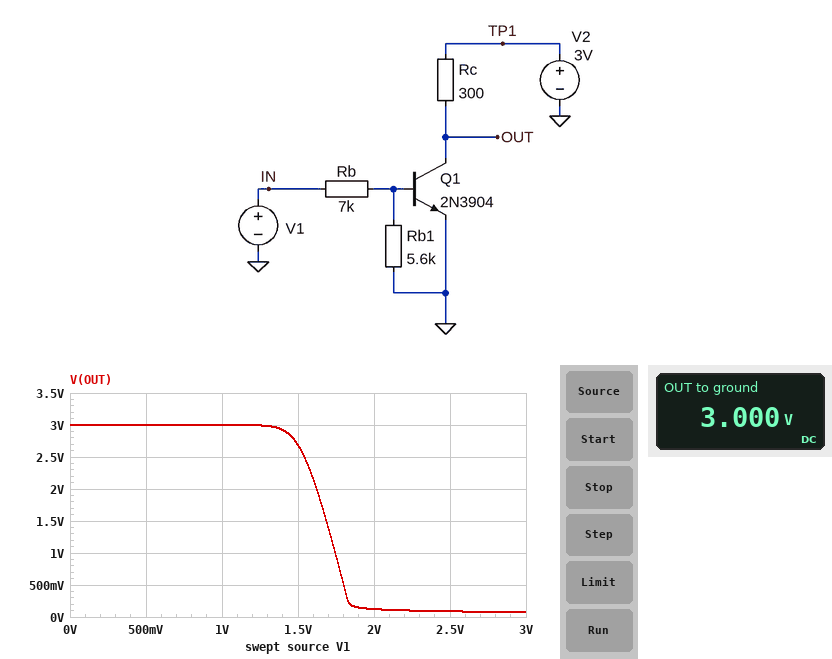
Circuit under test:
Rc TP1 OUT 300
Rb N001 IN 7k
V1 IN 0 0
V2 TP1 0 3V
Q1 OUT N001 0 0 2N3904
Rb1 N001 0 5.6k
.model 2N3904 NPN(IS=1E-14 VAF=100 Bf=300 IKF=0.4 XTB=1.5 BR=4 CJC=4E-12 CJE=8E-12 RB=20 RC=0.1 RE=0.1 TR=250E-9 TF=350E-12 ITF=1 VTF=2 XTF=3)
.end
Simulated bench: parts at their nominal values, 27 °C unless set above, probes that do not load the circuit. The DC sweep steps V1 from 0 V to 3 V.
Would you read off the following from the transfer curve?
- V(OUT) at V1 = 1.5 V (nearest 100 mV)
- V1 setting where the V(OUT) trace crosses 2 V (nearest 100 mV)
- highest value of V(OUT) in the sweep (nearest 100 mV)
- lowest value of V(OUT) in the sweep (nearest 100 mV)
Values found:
2.7 V
1.6 V
3.0 V
100 mV
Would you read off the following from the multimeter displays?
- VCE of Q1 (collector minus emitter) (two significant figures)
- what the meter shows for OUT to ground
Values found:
3.0 V
3.000 V
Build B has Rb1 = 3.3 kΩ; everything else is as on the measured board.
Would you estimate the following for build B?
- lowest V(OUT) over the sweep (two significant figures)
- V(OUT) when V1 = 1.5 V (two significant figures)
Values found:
94 mV
3.0 V
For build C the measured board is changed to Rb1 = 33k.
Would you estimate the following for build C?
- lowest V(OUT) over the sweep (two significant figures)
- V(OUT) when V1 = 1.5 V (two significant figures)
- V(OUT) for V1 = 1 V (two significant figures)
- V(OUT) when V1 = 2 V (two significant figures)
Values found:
64 mV
100 mV
1.1 V
81 mV
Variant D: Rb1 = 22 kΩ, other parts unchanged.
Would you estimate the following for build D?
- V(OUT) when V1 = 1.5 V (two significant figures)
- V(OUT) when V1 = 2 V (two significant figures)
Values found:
110 mV
83 mV
